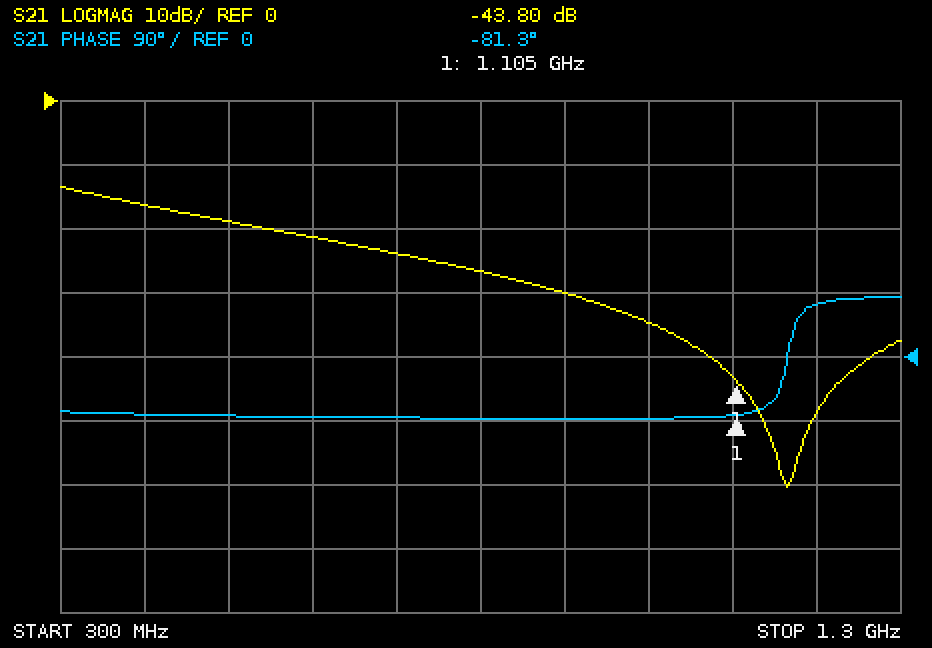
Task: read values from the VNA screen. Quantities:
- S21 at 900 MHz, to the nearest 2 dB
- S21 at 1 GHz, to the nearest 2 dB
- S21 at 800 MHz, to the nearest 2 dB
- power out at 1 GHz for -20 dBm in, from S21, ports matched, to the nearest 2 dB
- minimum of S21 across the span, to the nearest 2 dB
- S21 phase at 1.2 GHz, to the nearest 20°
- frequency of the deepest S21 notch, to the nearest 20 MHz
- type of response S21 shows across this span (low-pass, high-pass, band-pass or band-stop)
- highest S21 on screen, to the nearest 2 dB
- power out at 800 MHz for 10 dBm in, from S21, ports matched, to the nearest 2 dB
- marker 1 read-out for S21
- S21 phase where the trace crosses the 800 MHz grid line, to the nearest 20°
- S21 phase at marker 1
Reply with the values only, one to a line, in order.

-30 dB
-34 dB
-26 dB
-54 dBm
-60 dB
80°
1.16 GHz
low-pass
-14 dB
-16 dBm
-43.80 dB
-80°
-81.3°
